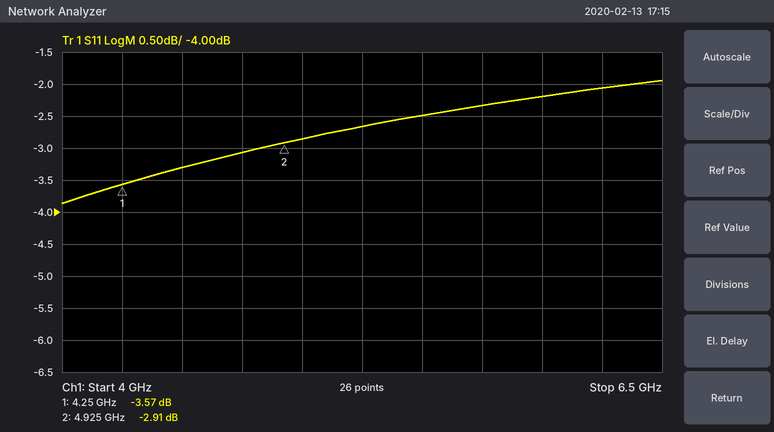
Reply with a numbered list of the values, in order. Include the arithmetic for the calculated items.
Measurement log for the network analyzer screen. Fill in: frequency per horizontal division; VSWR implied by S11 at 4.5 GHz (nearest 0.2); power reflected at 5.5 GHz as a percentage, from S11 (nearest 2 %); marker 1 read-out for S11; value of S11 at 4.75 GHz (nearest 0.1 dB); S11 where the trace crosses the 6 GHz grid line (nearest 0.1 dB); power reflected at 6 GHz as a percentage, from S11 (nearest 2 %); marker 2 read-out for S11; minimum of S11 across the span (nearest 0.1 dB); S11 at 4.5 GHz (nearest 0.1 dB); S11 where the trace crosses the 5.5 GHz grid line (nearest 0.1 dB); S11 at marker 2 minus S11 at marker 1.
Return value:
1. 250 MHz
2. |Γ| = 10^(-3.3/20) = 0.6839; VSWR = (1 + 0.6839)/(1 − 0.6839) ≈ 5.33, so 5.4 to the nearest 0.2
3. 10^(-2.5/10) ≈ 56 %
4. -3.57 dB
5. -3.1 dB
6. -2.2 dB
7. 10^(-2.2/10) ≈ 60 %
8. -2.91 dB
9. -3.9 dB
10. -3.3 dB
11. -2.5 dB
12. -2.91 − (-3.57) = 0.66 dB
